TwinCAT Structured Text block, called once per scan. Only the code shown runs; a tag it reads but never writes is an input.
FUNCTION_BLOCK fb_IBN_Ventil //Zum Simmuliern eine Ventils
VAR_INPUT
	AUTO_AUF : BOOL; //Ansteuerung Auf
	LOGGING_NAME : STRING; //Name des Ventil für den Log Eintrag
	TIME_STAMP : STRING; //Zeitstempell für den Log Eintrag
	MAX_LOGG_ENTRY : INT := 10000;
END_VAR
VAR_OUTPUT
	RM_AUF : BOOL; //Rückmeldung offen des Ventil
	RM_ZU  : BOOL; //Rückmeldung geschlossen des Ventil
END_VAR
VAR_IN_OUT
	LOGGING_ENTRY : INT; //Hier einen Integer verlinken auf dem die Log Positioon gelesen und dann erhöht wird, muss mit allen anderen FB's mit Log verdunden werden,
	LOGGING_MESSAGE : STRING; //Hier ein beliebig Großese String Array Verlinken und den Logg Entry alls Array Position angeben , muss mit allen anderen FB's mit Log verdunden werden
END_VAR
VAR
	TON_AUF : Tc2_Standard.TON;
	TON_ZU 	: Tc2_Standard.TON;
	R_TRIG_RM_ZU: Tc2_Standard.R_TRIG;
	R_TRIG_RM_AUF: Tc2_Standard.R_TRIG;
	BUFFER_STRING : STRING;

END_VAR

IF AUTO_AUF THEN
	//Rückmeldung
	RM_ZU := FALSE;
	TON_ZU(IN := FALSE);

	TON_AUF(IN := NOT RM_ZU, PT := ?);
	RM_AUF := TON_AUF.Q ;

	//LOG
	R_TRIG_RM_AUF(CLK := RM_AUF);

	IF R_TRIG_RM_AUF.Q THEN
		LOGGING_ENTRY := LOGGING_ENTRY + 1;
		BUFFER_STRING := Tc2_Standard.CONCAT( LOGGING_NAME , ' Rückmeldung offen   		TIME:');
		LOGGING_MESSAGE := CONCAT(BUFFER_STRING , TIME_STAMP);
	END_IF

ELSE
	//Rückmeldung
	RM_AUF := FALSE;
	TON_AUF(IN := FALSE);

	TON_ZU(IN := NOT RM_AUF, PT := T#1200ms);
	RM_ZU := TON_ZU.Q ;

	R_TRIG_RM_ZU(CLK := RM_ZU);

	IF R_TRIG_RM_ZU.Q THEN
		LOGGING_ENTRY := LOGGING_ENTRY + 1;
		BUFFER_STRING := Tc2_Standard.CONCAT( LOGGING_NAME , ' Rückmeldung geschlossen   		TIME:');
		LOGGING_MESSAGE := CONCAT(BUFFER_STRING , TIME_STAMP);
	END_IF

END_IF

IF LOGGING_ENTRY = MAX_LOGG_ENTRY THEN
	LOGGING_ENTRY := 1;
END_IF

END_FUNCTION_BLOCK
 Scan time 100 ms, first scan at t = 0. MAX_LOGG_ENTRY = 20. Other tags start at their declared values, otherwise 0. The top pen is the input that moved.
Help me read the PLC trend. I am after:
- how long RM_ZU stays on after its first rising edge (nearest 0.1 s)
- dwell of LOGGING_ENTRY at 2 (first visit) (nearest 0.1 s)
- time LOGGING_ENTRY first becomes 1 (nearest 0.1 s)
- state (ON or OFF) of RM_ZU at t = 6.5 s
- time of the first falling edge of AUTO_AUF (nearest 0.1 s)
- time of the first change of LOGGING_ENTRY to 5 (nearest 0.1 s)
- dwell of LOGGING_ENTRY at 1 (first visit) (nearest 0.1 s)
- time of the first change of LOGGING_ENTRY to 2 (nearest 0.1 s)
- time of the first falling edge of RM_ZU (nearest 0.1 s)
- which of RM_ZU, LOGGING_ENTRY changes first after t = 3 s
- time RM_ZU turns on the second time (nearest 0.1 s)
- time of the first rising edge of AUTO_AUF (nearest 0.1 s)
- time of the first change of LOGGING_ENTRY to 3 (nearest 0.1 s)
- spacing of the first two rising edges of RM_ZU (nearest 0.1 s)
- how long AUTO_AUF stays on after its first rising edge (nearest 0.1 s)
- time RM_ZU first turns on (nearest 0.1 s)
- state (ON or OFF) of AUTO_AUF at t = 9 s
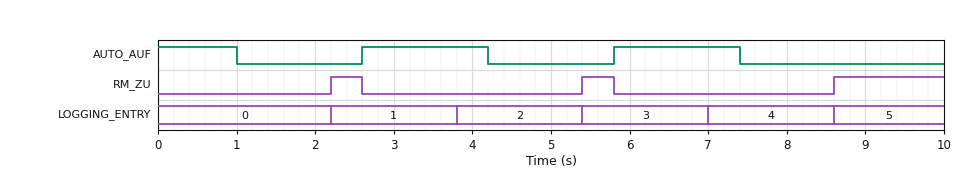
0.4 s
1.6 s
2.2 s
OFF
1.0 s
8.6 s
1.6 s
3.8 s
2.6 s
LOGGING_ENTRY
5.4 s
2.6 s
5.4 s
3.2 s
1.6 s
2.2 s
OFF
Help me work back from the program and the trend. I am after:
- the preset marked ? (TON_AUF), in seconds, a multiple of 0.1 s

1.2 s
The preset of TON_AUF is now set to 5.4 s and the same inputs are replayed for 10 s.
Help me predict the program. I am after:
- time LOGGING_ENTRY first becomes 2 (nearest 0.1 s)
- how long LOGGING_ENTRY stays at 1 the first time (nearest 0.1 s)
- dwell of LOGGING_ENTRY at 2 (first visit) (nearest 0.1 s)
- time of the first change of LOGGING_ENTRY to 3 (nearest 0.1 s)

5.4 s
3.2 s
3.2 s
8.6 s
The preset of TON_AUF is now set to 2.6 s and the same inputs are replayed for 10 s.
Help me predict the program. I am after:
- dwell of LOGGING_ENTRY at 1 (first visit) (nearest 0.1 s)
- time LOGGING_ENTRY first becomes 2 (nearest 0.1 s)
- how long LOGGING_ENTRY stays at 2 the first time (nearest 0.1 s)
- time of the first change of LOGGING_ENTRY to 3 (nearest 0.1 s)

3.2 s
5.4 s
3.2 s
8.6 s
